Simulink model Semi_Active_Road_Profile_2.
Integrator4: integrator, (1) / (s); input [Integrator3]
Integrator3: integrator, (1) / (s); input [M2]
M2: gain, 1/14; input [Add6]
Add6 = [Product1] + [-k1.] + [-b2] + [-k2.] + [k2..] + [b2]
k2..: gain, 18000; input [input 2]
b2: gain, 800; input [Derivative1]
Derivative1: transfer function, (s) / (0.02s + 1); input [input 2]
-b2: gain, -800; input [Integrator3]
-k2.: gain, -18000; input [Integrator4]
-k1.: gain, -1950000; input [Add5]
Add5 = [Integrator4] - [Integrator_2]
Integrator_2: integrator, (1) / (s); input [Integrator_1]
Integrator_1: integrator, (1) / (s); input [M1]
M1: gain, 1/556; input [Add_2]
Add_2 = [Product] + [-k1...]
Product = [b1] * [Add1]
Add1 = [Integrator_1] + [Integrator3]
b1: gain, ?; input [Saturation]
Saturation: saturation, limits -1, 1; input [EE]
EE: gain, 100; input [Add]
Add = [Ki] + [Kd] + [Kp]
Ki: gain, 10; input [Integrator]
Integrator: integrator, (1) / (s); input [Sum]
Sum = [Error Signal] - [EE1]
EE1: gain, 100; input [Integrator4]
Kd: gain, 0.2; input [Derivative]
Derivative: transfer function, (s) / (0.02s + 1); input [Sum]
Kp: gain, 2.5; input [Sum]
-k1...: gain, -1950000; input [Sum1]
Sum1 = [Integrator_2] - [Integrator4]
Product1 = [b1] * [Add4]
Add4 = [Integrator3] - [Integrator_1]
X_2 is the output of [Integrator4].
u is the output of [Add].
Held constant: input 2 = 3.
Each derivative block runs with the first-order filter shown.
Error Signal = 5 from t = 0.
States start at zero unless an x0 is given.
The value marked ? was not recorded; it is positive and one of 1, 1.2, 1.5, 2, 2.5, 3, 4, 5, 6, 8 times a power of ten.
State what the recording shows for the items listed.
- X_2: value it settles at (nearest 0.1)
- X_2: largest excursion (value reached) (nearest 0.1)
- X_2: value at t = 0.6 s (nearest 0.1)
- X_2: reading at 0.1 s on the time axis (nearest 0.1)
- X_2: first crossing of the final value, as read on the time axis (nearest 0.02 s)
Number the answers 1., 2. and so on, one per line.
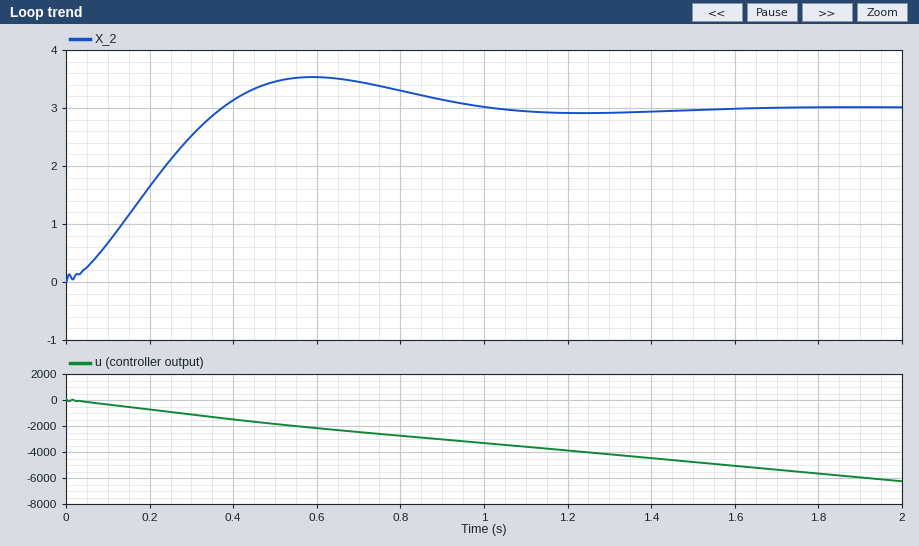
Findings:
1. 3.0
2. 3.5
3. 3.5
4. 0.7
5. 0.38 s
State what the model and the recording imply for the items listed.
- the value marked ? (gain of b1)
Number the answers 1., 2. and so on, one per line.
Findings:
1. 1200
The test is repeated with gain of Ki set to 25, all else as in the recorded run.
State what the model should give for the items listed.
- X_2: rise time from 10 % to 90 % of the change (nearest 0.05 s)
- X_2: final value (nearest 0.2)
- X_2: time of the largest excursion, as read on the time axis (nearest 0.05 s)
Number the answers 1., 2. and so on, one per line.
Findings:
1. 0.25 s
2. 3.0
3. 0.60 s
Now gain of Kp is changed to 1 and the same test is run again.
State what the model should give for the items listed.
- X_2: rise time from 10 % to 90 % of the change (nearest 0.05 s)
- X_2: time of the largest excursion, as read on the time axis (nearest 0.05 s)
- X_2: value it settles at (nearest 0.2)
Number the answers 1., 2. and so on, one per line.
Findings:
1. 0.25 s
2. 0.60 s
3. 3.0
